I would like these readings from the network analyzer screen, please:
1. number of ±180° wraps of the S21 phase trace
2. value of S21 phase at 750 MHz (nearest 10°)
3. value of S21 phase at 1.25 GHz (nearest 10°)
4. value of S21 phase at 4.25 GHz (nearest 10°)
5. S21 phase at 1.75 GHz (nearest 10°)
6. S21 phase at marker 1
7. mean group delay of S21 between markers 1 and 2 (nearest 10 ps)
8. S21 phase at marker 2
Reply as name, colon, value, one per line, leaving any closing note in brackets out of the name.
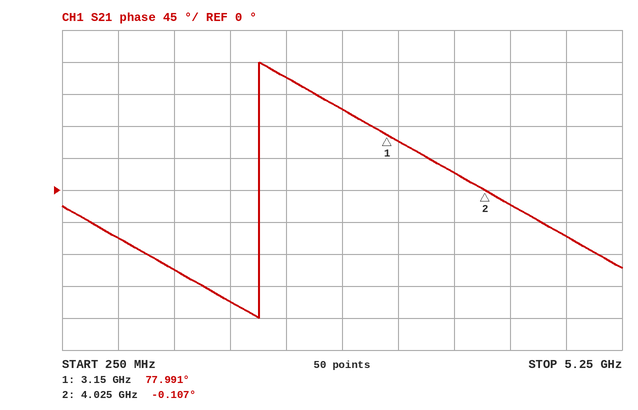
number of ±180° wraps of the S21 phase trace: 1
value of S21 phase at 750 MHz: -70°
value of S21 phase at 1.25 GHz: -110°
value of S21 phase at 4.25 GHz: -20°
S21 phase at 1.75 GHz: -160°
S21 phase at marker 1: 77.991°
mean group delay of S21 between markers 1 and 2: 250 ps
S21 phase at marker 2: -0.107°
